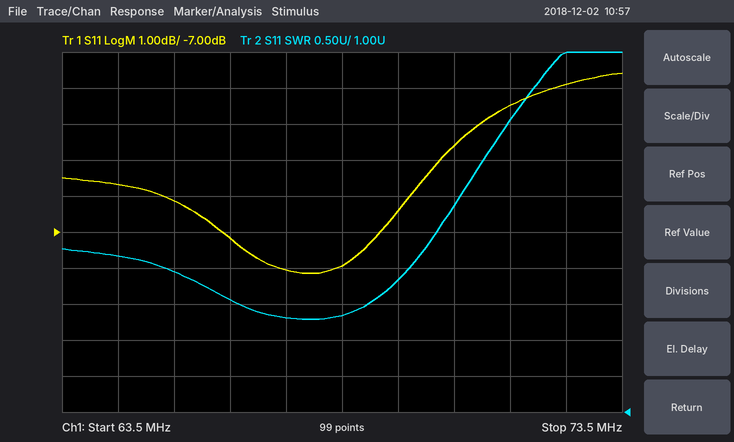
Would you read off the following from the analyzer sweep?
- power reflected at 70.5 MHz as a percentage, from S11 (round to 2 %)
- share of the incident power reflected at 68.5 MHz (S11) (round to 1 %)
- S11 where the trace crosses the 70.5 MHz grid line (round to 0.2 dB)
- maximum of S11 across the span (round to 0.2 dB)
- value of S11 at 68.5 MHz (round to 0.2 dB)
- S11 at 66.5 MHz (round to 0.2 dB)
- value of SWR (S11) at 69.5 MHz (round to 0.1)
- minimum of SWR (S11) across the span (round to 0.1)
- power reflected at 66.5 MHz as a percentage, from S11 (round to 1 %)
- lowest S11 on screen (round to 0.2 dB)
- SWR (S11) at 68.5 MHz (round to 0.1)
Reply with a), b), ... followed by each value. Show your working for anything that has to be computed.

a) 10^(-4.6/10) ≈ 34.7 %, so 34 % to the nearest 2 %
b) 10^(-8/10) ≈ 16 %
c) -4.6 dB
d) -2.6 dB
e) -8.0 dB
f) -7.2 dB
g) 2.8
h) 2.3
i) 10^(-7.2/10) ≈ 19 %
j) -8.2 dB
k) 2.3
